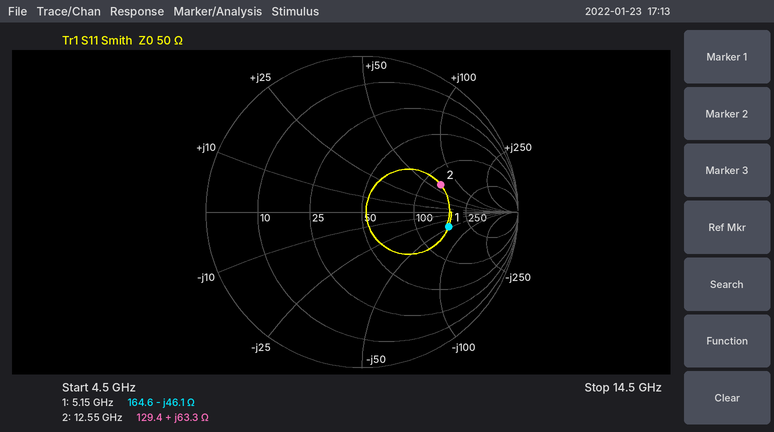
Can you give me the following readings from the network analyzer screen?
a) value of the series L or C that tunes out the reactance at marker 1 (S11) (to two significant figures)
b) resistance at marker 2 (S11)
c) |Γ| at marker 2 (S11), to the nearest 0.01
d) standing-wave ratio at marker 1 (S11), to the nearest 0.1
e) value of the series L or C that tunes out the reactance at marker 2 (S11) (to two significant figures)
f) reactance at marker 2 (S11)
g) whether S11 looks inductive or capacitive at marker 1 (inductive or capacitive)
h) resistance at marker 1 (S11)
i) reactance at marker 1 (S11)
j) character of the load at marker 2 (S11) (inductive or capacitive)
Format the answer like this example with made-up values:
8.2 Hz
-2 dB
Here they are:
1.4 nH
129.4 Ω
0.53
3.6
200 fF
+63.3 Ω
capacitive
164.6 Ω
-46.1 Ω
inductive
